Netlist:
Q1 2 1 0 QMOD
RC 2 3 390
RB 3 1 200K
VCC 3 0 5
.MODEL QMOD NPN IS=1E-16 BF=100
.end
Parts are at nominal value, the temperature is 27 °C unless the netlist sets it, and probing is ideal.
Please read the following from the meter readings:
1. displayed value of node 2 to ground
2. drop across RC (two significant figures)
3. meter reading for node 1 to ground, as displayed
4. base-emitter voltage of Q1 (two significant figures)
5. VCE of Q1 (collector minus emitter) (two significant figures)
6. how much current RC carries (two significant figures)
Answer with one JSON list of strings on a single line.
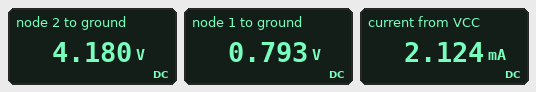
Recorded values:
["4.180 V", "820 mV", "0.793 V", "790 mV", "4.2 V", "2.1 mA"]
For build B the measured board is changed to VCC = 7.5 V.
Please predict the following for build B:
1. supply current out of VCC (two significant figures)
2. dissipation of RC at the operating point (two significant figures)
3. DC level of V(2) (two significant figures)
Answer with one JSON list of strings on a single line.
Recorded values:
["3.4 mA", "4.4 mW", "6.2 V"]
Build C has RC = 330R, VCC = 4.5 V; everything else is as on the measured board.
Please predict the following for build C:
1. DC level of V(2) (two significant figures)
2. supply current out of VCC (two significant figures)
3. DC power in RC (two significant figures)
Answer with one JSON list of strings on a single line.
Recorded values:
["3.9 V", "1.9 mA", "1.1 mW"]
